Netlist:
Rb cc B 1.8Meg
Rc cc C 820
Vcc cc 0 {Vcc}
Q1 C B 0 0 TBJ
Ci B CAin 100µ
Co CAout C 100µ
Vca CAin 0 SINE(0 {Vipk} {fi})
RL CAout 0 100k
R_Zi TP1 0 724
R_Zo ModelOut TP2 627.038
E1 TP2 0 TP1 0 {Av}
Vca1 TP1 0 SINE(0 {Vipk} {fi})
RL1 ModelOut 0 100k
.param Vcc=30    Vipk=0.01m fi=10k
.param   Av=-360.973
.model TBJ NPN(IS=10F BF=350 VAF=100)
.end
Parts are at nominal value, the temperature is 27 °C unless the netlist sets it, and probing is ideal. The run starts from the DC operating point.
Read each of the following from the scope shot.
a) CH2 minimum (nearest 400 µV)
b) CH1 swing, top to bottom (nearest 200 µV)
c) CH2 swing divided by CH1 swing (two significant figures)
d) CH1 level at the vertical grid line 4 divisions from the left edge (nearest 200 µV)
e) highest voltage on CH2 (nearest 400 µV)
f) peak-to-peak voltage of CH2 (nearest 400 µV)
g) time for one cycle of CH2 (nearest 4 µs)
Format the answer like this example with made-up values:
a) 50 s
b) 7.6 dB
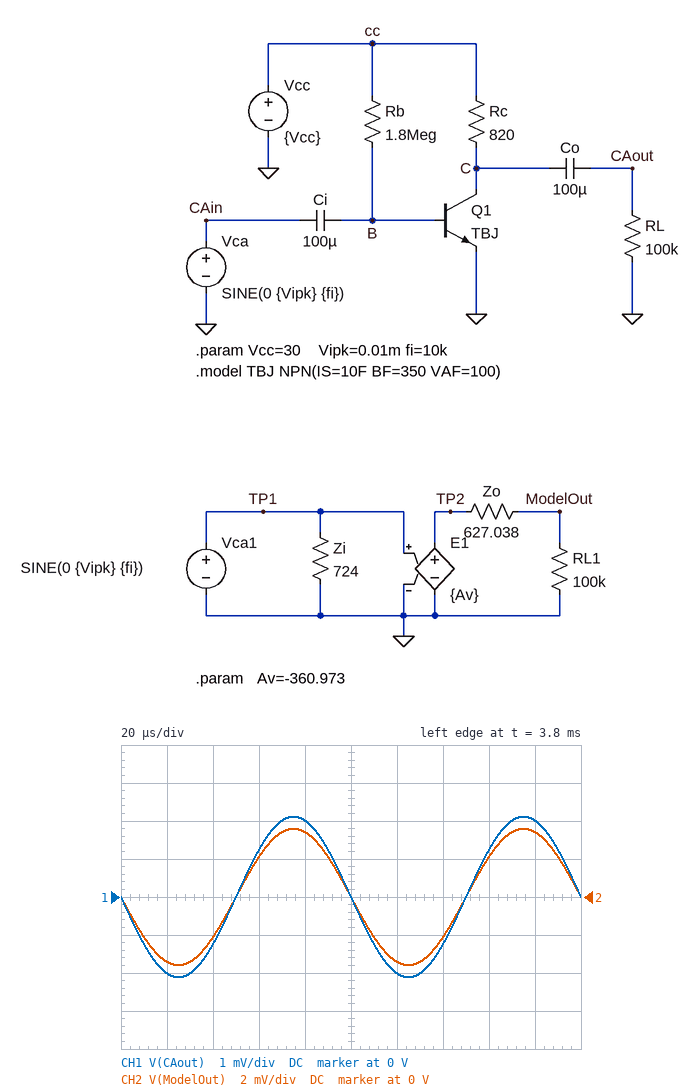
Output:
a) -3.6 mV
b) 4.2 mV
c) 1.7
d) 2.0 mV
e) 3.6 mV
f) 7.2 mV
g) 100 µs
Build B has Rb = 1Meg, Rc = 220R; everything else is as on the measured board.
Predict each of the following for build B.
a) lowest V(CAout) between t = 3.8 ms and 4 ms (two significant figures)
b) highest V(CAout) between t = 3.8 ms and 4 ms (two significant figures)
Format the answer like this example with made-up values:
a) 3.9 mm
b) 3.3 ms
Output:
a) -1.1 mV
b) 1.1 mV
